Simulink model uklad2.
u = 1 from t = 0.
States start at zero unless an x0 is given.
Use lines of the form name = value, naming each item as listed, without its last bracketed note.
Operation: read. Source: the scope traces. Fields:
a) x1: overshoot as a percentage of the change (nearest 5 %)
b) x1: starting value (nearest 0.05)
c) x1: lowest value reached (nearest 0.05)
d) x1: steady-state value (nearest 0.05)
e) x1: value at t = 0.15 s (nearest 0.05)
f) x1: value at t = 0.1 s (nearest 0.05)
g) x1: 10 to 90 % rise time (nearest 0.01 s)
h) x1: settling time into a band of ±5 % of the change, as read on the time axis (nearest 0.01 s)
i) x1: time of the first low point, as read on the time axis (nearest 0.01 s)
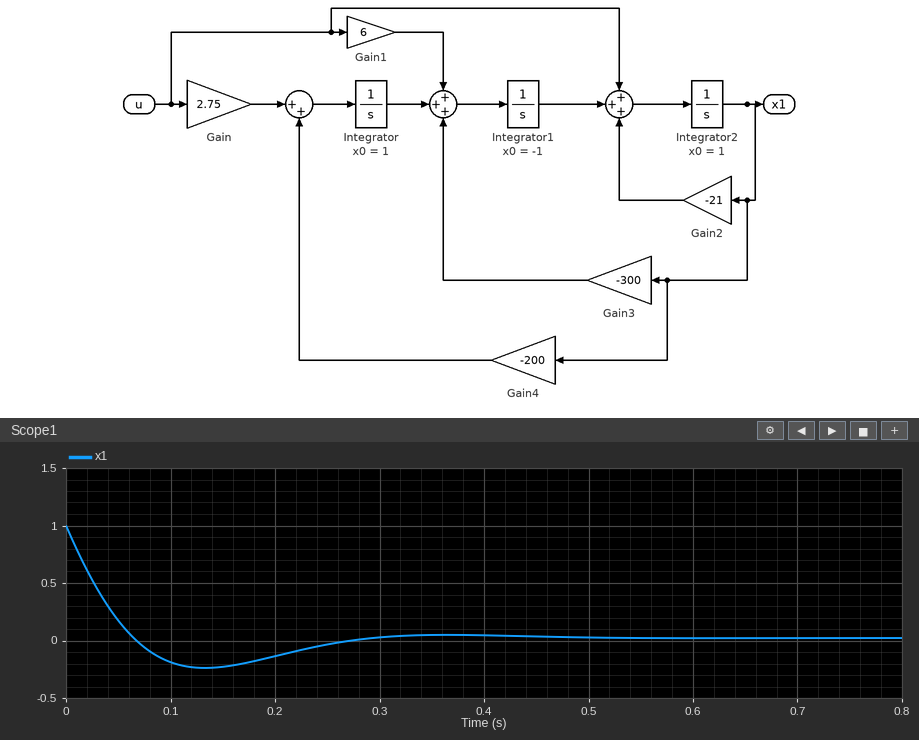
x1: overshoot as a percentage of the change = 25 %
x1: starting value = 1.00
x1: lowest value reached = -0.25
x1: steady-state value = 0.00
x1: value at t = 0.15 s = -0.25
x1: value at t = 0.1 s = -0.20
x1: 10 to 90 % rise time = 0.05 s
x1: settling time into a band of ±5 % of the change, as read on the time axis = 0.25 s
x1: time of the first low point, as read on the time axis = 0.13 s
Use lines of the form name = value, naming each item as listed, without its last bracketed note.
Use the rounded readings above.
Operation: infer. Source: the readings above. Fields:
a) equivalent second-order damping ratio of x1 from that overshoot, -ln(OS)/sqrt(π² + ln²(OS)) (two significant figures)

equivalent second-order damping ratio of x1 from that overshoot, -ln(OS)/sqrt(π² + ln²(OS)) = 0.40
